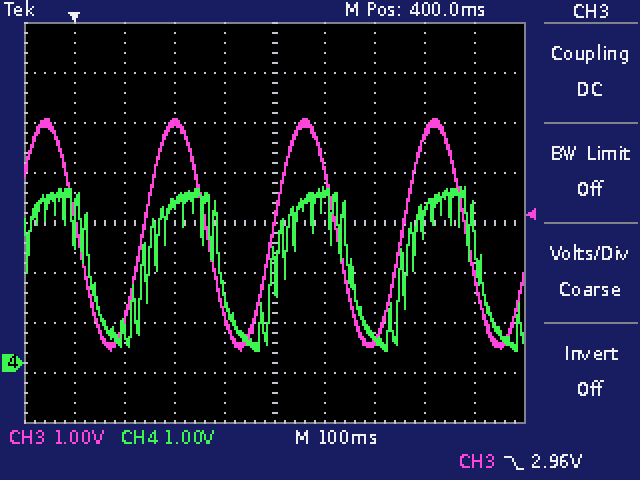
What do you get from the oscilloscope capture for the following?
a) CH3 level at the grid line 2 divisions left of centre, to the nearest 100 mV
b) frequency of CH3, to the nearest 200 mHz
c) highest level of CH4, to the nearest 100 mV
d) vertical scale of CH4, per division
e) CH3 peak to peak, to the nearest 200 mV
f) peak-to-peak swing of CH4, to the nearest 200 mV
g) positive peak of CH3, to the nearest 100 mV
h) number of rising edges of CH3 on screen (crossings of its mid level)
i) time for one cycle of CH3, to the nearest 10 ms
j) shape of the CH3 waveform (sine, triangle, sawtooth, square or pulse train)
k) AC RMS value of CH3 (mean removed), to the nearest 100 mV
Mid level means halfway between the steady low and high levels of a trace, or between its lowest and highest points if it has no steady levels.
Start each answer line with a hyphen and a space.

- 4.8 V
- 3.8 Hz
- 3.5 V
- 1 V
- 4.6 V
- 3.2 V
- 4.9 V
- 3
- 260 ms
- sine
- 1.6 V
